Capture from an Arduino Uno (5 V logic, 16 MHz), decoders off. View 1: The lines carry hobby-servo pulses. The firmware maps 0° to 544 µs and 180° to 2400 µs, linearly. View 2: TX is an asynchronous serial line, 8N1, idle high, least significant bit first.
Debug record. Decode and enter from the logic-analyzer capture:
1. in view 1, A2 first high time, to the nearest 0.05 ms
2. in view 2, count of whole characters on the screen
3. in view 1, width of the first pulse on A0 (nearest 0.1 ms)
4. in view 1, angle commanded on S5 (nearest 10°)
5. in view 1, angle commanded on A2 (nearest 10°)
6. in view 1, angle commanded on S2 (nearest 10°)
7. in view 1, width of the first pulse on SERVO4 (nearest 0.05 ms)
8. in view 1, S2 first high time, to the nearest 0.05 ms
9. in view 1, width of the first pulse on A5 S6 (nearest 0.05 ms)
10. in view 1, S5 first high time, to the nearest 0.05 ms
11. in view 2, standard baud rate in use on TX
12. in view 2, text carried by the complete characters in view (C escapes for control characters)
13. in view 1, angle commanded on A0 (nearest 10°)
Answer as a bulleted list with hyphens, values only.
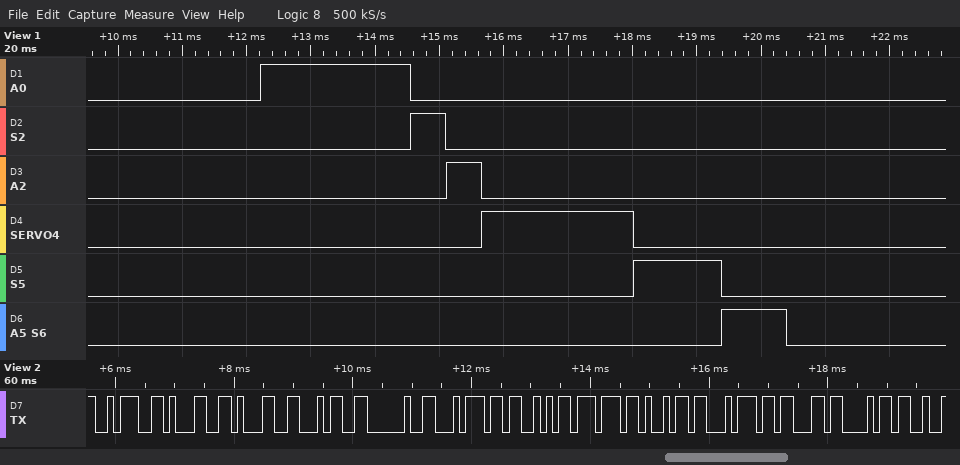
- 0.55 ms
- 12
- 2.3 ms
- 80°
- 0°
- 0°
- 2.35 ms
- 0.55 ms
- 1.00 ms
- 1.35 ms
- 9600 baud
- ":114 tSwitch"
- 170°
